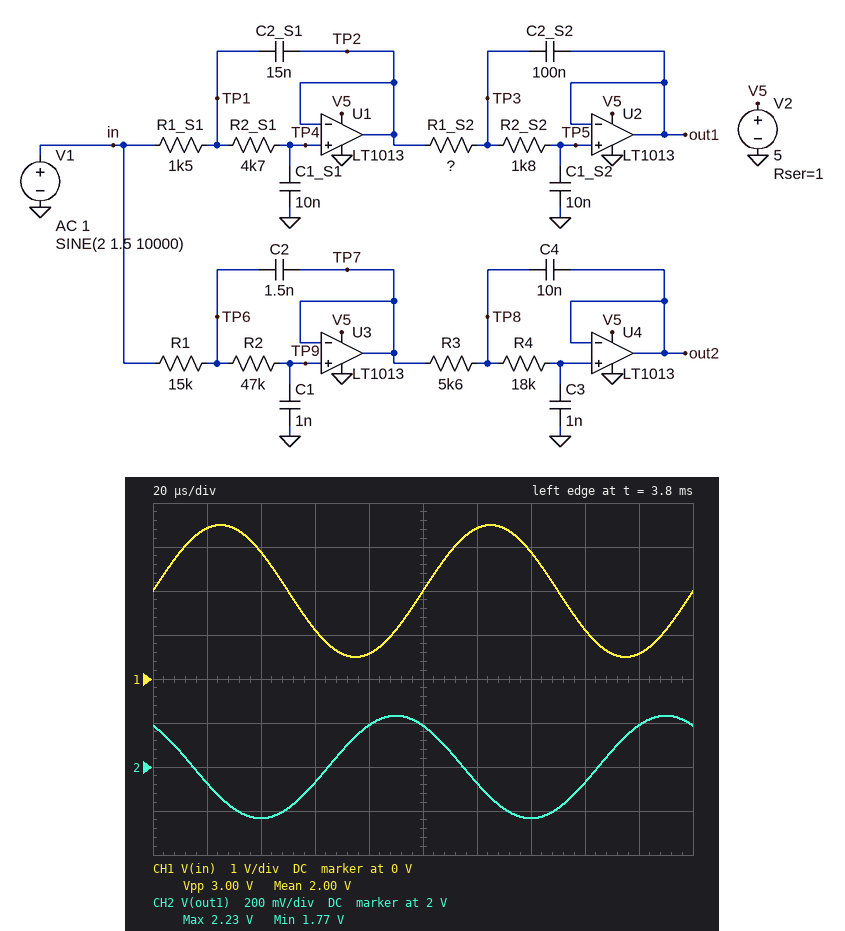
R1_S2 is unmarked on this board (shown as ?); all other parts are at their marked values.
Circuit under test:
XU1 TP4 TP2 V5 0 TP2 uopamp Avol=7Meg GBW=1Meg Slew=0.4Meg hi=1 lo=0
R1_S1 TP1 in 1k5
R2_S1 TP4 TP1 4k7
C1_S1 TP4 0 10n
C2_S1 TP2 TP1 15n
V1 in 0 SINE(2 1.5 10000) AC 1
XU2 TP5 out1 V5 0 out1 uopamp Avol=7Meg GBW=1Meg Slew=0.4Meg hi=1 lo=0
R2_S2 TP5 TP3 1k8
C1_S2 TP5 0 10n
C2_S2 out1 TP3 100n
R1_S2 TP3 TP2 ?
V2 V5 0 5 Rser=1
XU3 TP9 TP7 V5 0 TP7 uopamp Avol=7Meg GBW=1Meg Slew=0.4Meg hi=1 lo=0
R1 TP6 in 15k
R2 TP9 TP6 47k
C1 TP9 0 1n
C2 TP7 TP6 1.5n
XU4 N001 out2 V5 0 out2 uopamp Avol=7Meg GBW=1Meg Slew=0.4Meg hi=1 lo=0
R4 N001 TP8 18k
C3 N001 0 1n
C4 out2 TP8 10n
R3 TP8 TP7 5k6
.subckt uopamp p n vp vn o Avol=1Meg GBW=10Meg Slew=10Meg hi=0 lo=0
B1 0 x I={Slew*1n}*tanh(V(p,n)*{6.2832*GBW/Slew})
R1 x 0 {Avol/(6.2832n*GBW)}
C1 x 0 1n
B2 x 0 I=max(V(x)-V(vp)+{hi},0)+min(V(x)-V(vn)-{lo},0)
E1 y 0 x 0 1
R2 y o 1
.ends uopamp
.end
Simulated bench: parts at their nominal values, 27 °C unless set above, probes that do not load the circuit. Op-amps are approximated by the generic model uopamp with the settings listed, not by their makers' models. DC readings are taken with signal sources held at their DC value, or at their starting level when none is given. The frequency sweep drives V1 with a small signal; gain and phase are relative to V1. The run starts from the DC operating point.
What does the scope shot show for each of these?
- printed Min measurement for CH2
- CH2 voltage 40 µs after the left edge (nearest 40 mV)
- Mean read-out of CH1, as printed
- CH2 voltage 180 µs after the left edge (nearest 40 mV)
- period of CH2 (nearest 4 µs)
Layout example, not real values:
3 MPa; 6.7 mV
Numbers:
1.77 V; 1.76 V; 2.00 V; 2.20 V; 100 µs
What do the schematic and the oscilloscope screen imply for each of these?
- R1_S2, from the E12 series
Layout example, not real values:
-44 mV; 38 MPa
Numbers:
180 Ω
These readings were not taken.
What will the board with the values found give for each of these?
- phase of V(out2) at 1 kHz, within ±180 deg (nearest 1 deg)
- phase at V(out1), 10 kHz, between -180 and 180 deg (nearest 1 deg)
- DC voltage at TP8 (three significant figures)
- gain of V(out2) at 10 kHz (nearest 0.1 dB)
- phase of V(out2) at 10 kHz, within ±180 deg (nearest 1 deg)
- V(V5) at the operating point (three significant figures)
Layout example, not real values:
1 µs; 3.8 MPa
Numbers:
-31 deg; 126 deg; 2.00 V; -24.6 dB; 76 deg; 5.00 V
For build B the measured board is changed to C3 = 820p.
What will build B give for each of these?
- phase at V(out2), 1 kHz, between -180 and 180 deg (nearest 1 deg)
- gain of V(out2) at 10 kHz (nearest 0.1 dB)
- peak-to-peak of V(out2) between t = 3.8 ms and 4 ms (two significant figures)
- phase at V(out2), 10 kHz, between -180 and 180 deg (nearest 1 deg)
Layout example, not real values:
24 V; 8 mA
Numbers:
-29 deg; -22.3 dB; 230 mV; 77 deg
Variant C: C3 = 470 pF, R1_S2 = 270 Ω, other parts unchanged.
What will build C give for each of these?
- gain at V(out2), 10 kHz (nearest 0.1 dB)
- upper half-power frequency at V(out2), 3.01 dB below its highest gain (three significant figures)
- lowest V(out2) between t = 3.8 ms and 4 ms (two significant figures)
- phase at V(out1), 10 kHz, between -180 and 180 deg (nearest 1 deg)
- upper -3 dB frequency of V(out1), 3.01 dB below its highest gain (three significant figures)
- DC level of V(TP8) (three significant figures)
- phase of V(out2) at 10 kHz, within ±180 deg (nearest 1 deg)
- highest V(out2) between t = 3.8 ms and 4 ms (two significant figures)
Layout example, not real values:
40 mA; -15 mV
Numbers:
-15.2 dB; 6.93 kHz; 1.7 V; 104 deg; 4.18 kHz; 2.00 V; 87 deg; 2.3 V
